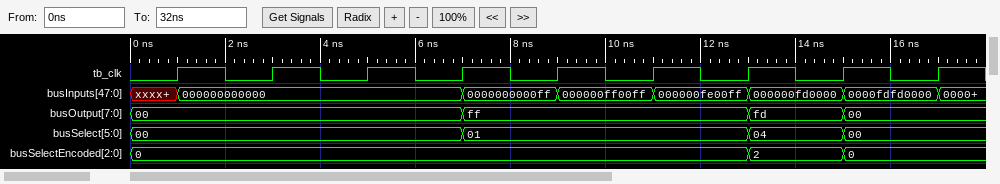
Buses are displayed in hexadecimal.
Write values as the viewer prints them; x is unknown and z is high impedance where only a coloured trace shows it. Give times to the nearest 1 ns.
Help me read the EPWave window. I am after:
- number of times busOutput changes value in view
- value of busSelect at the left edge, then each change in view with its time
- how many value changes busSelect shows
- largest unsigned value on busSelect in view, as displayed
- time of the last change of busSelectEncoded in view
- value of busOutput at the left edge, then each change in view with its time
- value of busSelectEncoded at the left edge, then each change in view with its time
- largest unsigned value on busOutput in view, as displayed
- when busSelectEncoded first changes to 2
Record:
3
00, 01 at 7 ns, 04 at 13 ns, 00 at 15 ns
3
04
15 ns
00, ff at 7 ns, fd at 13 ns, 00 at 15 ns
0, 2 at 13 ns, 0 at 15 ns
ff
13 ns
